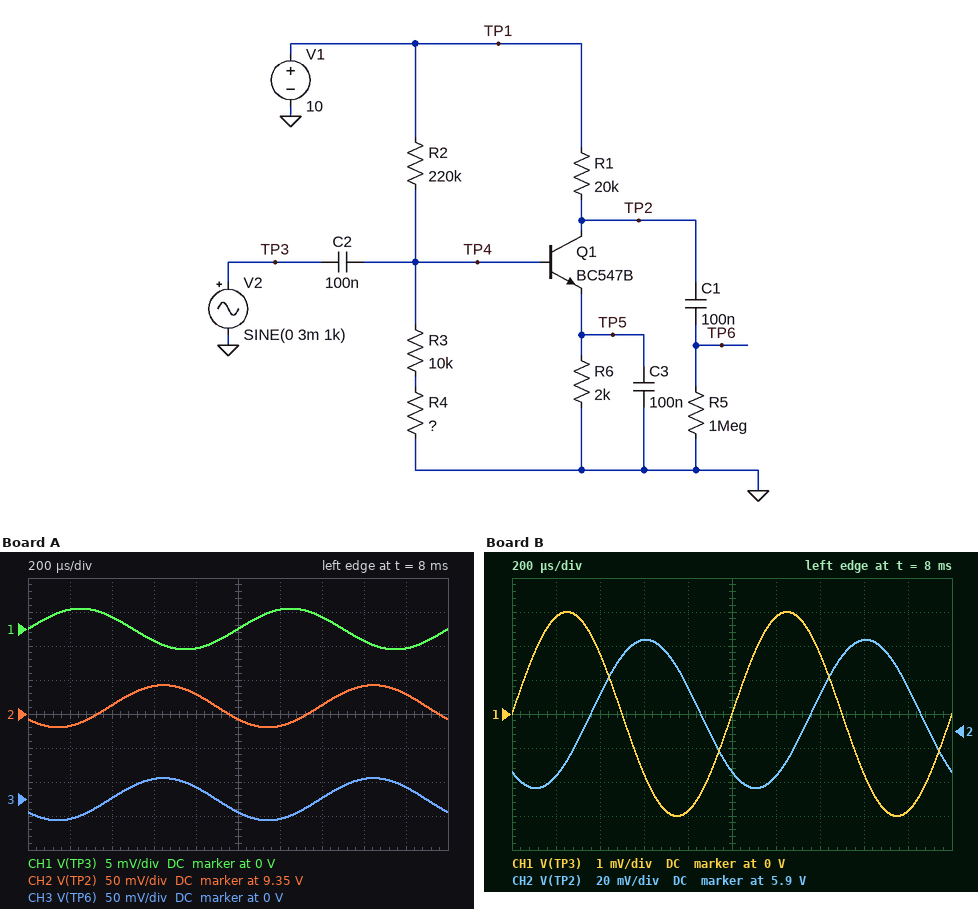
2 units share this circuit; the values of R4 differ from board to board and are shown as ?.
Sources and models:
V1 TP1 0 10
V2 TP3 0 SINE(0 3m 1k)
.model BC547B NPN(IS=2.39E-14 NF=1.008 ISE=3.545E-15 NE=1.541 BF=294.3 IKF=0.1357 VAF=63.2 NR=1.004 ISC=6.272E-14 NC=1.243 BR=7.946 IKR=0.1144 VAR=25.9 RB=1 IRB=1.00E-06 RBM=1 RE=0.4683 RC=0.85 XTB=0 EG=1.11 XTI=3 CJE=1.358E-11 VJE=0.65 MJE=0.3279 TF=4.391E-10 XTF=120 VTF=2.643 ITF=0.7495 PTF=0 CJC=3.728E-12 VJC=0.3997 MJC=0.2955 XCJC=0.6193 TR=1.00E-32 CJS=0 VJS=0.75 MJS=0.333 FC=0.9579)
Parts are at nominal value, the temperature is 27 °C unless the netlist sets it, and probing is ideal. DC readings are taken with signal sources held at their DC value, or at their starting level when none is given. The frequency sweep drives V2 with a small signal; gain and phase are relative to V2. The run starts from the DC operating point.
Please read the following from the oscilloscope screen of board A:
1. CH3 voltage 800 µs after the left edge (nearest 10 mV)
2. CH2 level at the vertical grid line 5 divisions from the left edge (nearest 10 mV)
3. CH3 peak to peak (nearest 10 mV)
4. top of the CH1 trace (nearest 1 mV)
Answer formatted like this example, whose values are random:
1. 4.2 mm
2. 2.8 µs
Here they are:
1. 20 mV
2. 9.34 V
3. 60 mV
4. 3 mV
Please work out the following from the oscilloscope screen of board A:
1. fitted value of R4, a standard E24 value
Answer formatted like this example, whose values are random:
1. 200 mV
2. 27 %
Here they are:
1. 4.3 kΩ
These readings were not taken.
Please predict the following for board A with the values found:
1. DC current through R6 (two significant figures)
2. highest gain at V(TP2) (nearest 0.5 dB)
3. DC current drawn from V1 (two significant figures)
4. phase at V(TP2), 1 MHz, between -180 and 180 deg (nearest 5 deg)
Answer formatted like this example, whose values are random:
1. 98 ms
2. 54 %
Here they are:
1. 32 µA
2. 27.5 dB
3. 75 µA
4. 170 deg
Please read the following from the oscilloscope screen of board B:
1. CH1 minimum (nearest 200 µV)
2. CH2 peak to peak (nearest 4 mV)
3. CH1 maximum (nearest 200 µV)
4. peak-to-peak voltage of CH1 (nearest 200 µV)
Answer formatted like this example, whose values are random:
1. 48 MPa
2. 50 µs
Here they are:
1. -3.0 mV
2. 88 mV
3. 3.0 mV
4. 6.0 mV
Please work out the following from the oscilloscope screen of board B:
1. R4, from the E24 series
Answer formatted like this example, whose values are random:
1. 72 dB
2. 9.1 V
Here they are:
1. 15 kΩ
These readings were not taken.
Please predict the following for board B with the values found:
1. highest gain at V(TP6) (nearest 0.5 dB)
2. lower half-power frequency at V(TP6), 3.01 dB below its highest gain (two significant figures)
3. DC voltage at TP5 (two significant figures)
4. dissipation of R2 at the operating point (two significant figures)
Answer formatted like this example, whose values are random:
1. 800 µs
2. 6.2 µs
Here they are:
1. 43.0 dB
2. 12 kHz
3. 410 mV
4. 370 µW
